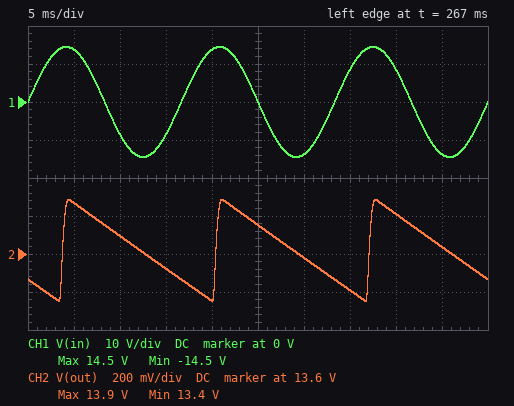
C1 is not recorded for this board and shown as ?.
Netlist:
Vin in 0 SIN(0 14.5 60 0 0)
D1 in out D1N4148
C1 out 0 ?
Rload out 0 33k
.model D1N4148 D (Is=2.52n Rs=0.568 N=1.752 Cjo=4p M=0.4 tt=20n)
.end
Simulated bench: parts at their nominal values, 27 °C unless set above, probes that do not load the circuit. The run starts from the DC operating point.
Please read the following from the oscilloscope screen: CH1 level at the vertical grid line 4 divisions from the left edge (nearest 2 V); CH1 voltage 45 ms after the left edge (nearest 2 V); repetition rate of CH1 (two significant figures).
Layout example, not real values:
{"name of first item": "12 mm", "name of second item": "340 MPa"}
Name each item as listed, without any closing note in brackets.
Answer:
{"CH1 level at the vertical grid line 4 divisions from the left edge": "14 V", "CH1 voltage 45 ms after the left edge": "-14 V", "repetition rate of CH1": "60 Hz"}
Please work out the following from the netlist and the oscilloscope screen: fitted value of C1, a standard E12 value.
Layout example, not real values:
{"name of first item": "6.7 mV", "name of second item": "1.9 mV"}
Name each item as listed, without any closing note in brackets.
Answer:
{"fitted value of C1, a standard E12 value": "12 µF"}
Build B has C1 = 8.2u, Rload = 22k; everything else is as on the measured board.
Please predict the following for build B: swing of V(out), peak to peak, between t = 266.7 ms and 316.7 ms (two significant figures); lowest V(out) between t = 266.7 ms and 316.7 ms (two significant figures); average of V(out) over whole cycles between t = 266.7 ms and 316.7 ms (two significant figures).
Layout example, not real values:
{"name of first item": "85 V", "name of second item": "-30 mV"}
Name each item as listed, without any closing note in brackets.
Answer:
{"swing of V(out), peak to peak, between t = 266.7 ms and 316.7 ms": "1.1 V", "lowest V(out) between t = 266.7 ms and 316.7 ms": "13 V", "average of V(out) over whole cycles between t = 266.7 ms and 316.7 ms": "13 V"}
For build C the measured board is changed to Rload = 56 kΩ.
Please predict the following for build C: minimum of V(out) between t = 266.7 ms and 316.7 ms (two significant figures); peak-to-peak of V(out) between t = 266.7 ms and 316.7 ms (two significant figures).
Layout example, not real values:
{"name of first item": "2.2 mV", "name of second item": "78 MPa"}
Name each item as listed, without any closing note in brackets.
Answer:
{"minimum of V(out) between t = 266.7 ms and 316.7 ms": "14 V", "peak-to-peak of V(out) between t = 266.7 ms and 316.7 ms": "320 mV"}
